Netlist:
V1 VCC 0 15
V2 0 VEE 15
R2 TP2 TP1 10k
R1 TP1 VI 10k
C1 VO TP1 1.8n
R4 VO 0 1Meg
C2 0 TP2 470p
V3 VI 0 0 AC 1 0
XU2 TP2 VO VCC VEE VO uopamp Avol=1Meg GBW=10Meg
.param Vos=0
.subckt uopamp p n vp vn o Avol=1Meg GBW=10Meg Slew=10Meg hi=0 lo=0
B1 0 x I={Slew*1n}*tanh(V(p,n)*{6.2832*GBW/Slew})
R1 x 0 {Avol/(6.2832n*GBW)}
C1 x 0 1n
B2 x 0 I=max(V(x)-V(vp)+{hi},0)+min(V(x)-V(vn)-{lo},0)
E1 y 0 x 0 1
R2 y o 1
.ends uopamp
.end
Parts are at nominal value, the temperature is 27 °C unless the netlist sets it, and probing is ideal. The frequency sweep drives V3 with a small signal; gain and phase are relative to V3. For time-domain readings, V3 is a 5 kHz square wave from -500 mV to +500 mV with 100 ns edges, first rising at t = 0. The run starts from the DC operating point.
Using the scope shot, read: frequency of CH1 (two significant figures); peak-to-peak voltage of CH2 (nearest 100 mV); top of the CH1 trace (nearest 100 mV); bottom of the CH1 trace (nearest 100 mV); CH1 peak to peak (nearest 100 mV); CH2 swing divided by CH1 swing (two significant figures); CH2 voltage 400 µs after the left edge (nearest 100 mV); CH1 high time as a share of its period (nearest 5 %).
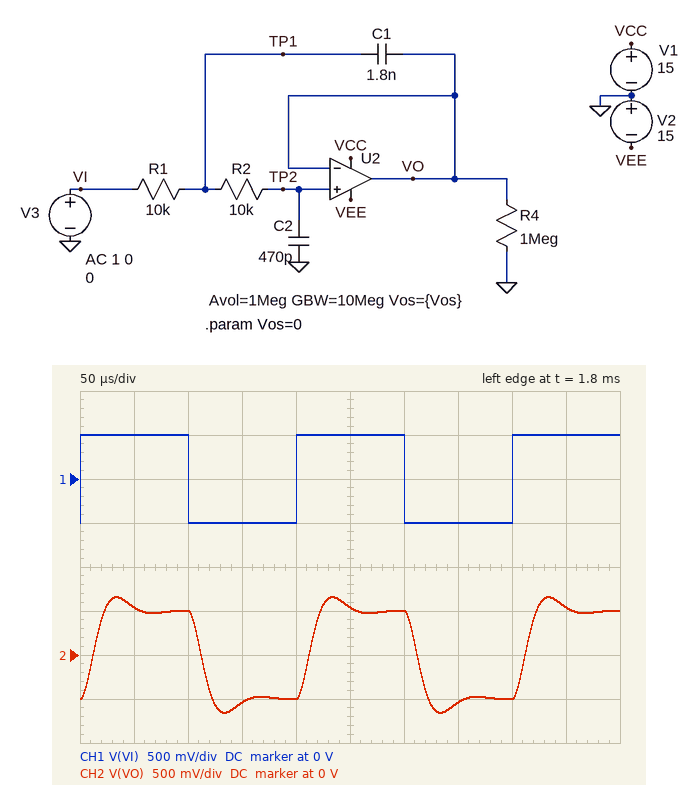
5.0 kHz
1.3 V
500 mV
-500 mV
1.0 V
1.3
-500 mV
50 %
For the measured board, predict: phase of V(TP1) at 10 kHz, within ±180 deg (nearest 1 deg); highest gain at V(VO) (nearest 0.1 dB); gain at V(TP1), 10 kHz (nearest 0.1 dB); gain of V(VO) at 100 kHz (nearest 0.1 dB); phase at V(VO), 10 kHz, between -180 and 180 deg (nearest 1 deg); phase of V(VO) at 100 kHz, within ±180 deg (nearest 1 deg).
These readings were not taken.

-25 deg
1.1 dB
1.4 dB
-30.4 dB
-42 deg
-170 deg
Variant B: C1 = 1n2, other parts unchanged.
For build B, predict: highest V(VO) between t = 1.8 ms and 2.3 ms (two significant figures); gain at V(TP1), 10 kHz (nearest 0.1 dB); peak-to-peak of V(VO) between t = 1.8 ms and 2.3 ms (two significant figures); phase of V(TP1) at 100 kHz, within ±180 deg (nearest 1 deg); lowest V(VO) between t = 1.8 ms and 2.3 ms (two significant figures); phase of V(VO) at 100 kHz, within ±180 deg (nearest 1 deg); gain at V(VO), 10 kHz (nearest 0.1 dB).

580 mV
0.6 dB
1.2 V
-93 deg
-580 mV
-165 deg
0.2 dB
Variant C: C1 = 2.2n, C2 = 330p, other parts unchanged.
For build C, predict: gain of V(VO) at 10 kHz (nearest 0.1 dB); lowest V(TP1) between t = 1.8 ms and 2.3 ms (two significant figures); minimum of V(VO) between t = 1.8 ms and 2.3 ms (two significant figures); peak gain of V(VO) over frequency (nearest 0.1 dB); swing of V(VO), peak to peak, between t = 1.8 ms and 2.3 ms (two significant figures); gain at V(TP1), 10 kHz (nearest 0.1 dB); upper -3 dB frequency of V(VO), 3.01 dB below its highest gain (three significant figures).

1.7 dB
-790 mV
-770 mV
2.9 dB
1.5 V
1.9 dB
22.2 kHz
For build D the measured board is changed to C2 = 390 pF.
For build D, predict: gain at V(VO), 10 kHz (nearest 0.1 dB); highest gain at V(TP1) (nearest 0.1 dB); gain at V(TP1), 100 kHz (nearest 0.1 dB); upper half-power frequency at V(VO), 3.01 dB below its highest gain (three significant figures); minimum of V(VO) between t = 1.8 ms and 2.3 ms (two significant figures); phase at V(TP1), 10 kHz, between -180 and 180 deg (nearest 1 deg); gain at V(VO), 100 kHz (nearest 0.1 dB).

1.2 dB
2.2 dB
-20.3 dB
22.4 kHz
-690 mV
-20 deg
-28.7 dB
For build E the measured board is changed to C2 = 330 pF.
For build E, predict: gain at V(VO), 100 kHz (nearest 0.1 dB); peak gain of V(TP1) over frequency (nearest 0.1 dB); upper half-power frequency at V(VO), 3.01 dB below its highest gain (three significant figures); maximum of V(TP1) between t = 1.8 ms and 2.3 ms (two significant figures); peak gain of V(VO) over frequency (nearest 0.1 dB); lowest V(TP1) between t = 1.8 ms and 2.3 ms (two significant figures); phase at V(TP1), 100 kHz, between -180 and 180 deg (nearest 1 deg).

-27.2 dB
2.7 dB
24.4 kHz
750 mV
2.2 dB
-750 mV
-105 deg
